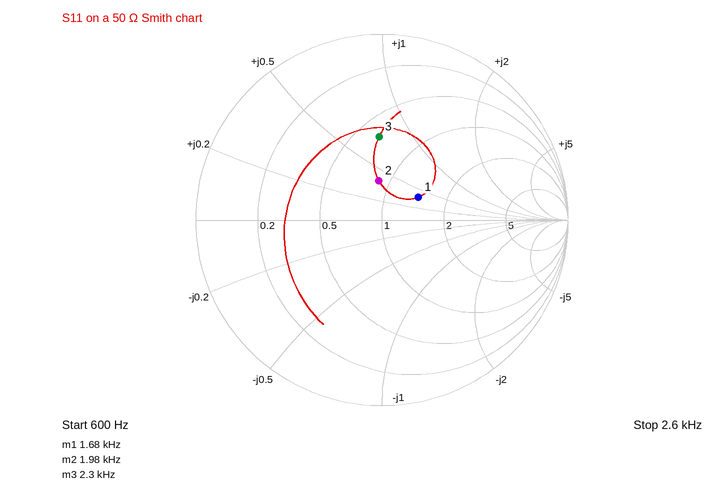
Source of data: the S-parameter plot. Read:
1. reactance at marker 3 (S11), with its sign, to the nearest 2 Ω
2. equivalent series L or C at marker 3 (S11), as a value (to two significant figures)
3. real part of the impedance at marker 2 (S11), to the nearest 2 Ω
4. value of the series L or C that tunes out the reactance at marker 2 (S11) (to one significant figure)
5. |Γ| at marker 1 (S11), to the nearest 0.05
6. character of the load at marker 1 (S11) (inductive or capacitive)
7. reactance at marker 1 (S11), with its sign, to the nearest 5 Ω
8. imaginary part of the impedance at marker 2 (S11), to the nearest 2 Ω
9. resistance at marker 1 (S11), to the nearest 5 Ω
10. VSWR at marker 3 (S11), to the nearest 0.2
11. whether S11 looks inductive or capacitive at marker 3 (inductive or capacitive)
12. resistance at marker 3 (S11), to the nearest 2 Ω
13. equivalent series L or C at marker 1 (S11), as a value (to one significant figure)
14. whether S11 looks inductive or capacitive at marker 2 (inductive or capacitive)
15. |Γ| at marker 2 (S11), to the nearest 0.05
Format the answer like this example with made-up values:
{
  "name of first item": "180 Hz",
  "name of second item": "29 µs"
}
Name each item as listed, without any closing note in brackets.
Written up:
{
  "reactance at marker 3 (S11), with its sign, to the nearest 2 Ω": "+36 Ω",
  "equivalent series L or C at marker 3 (S11), as a value": "2.5 mH",
  "real part of the impedance at marker 2 (S11), to the nearest 2 Ω": "44 Ω",
  "value of the series L or C that tunes out the reactance at marker 2 (S11)": "4 µF",
  "|Γ| at marker 1 (S11), to the nearest 0.05": "0.25",
  "character of the load at marker 1 (S11)": "inductive",
  "reactance at marker 1 (S11), with its sign, to the nearest 5 Ω": "+20 Ω",
  "imaginary part of the impedance at marker 2 (S11), to the nearest 2 Ω": "+20 Ω",
  "resistance at marker 1 (S11), to the nearest 5 Ω": "70 Ω",
  "VSWR at marker 3 (S11), to the nearest 0.2": "2.6",
  "whether S11 looks inductive or capacitive at marker 3": "inductive",
  "resistance at marker 3 (S11), to the nearest 2 Ω": "32 Ω",
  "equivalent series L or C at marker 1 (S11), as a value": "2 mH",
  "whether S11 looks inductive or capacitive at marker 2": "inductive",
  "|Γ| at marker 2 (S11), to the nearest 0.05": "0.20"
}
